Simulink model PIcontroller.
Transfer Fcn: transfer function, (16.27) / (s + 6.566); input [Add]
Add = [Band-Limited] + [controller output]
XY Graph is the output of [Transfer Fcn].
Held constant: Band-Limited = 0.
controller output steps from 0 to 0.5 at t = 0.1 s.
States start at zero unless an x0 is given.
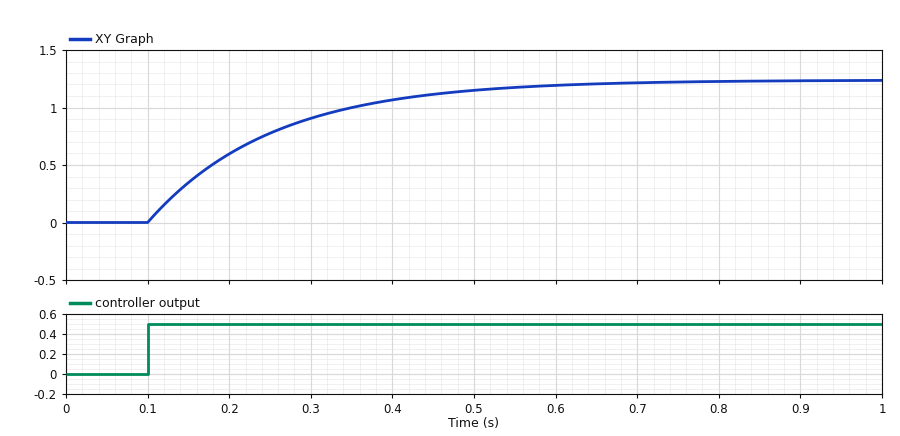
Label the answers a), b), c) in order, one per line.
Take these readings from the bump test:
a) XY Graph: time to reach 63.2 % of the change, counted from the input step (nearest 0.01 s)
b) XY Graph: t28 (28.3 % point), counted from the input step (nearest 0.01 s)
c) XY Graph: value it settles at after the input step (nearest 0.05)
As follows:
a) 0.15 s
b) 0.05 s
c) 1.25
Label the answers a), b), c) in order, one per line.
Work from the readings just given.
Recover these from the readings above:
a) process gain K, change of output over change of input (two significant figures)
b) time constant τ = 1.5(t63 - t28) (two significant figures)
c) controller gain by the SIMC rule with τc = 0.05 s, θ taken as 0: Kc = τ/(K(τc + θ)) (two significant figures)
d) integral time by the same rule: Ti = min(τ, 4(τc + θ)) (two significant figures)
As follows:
a) 2.5
b) 0.15 s
c) 1.2
d) 0.15 s
